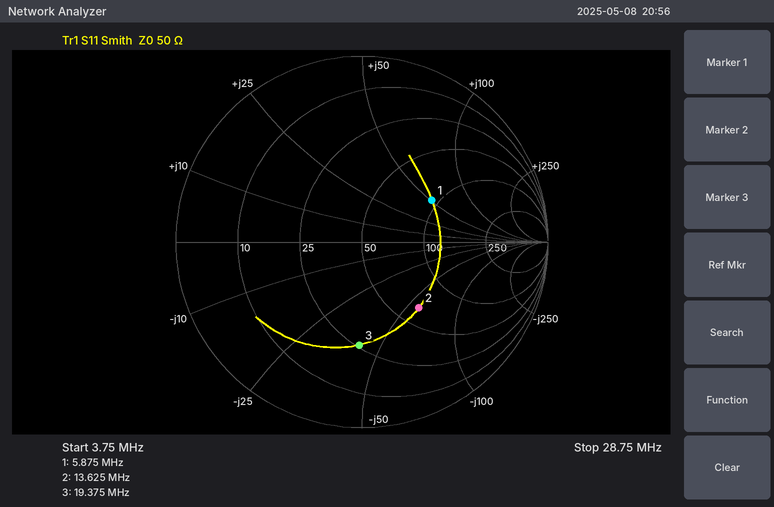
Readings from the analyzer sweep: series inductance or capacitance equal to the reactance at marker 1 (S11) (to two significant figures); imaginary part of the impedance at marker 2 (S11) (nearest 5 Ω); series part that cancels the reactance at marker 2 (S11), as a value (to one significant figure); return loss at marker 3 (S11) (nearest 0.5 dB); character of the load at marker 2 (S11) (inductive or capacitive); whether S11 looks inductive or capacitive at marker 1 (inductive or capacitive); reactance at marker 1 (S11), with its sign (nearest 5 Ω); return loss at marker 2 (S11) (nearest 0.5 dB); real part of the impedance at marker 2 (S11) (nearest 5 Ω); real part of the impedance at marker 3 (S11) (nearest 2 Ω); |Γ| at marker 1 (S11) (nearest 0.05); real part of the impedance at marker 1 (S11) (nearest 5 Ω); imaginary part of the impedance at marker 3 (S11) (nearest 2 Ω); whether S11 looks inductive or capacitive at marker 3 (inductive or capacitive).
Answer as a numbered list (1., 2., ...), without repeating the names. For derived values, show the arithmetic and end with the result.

1. L = 50 Ω/(2π × 5.875 MHz) ≈ 1.4 µH
2. -60 Ω
3. L = 60 Ω/(2π × 13.625 MHz) ≈ 701 nH, so 700 nH to one significant figure
4. 5.0 dB
5. capacitive
6. inductive
7. +50 Ω
8. 6.5 dB
9. 65 Ω
10. 26 Ω
11. 0.45
12. 90 Ω
13. -42 Ω
14. capacitive
